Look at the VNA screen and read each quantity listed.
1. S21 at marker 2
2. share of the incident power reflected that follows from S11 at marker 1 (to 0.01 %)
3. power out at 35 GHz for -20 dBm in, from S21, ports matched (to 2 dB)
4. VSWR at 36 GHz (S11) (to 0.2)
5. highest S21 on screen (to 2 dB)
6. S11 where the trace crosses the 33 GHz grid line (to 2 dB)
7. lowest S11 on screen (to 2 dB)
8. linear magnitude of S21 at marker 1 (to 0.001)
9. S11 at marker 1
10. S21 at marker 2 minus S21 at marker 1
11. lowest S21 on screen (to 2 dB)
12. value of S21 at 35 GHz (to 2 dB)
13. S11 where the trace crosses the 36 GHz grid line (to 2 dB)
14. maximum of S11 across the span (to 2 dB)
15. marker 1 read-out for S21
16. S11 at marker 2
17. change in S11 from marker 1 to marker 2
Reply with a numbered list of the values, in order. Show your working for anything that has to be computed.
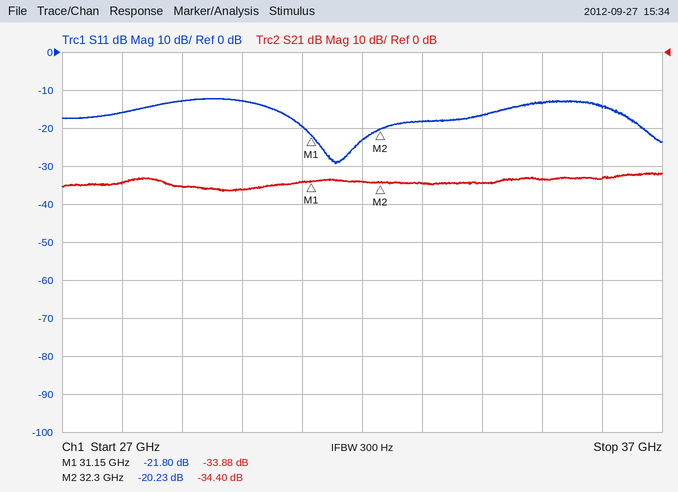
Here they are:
1. -34.40 dB
2. 10^(-21.8/10) ≈ 0.66 %
3. -20 dBm + (-34 dB) = -54 dBm
4. |Γ| = 10^(-14/20) = 0.1995; VSWR = (1 + 0.1995)/(1 − 0.1995) ≈ 1.50, so 1.4 to the nearest 0.2
5. -32 dB
6. -18 dB
7. -30 dB
8. 10^(-33.88/20) ≈ 0.020
9. -21.80 dB
10. -34.4 − (-33.88) = -0.52 dB
11. -36 dB
12. -34 dB
13. -14 dB
14. -12 dB
15. -33.88 dB
16. -20.23 dB
17. -20.23 − (-21.8) = 1.57 dB
